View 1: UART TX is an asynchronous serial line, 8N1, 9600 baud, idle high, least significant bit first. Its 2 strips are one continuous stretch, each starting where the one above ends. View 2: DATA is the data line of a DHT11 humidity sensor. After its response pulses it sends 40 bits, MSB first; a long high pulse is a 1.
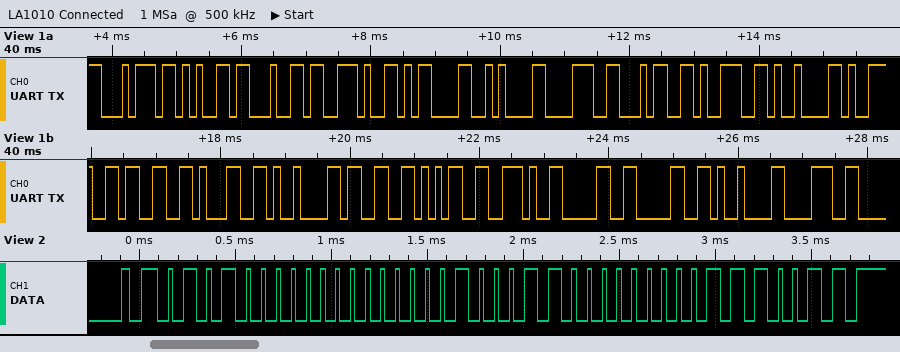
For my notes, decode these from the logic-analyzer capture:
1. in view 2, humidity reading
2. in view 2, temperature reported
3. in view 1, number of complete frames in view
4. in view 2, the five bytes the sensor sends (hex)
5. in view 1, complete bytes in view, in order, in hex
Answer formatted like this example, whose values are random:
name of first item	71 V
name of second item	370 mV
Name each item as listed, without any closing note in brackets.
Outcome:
in view 2, humidity reading	80 %
in view 2, temperature reported	35.0 °C
in view 1, number of complete frames in view	21
in view 2, the five bytes the sensor sends	50 00 23 00 73
in view 1, complete bytes in view, in order, in hex	74 65 64 2E 0D 0A 38 34 39 09 39 33 31 09 33 35 2E 30 30 09 38
